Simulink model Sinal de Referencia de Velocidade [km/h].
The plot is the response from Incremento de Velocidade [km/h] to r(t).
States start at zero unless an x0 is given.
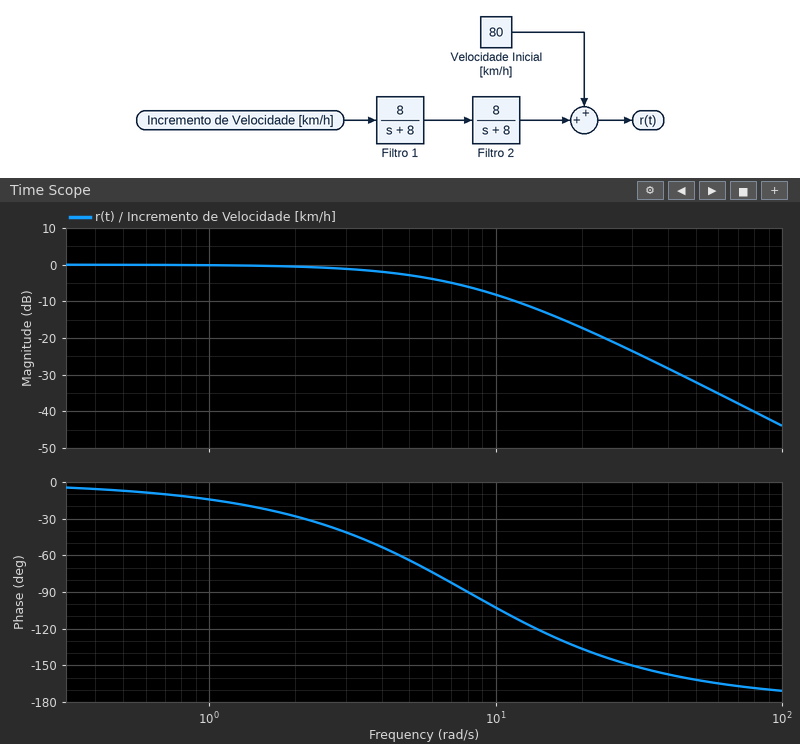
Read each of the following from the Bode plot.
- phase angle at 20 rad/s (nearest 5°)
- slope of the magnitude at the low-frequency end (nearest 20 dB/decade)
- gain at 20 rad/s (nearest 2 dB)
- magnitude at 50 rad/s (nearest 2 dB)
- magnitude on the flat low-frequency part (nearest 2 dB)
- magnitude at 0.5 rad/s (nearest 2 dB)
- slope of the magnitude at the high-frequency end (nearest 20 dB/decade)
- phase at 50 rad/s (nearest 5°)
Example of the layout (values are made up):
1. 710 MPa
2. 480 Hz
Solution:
1. -135°
2. 0 dB/decade
3. -18 dB
4. -32 dB
5. 0 dB
6. 0 dB
7. -40 dB/decade
8. -160°
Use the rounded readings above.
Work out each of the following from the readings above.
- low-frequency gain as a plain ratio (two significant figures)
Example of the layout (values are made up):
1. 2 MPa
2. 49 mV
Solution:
1. 1.0
